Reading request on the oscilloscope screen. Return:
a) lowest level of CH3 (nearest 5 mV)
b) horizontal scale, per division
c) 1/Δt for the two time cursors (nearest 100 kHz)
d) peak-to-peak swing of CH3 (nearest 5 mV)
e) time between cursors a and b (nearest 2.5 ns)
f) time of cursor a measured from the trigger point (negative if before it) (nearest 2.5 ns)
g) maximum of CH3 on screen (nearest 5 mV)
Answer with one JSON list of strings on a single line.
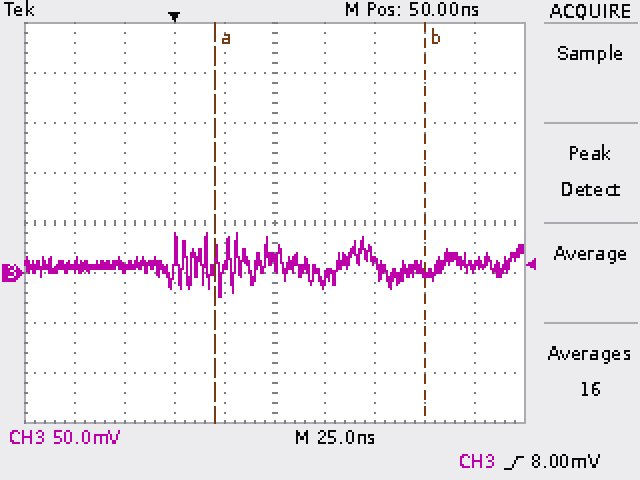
["-25 mV", "25 ns", "9.5 MHz", "65 mV", "105.0 ns", "+20.0 ns", "40 mV"]
